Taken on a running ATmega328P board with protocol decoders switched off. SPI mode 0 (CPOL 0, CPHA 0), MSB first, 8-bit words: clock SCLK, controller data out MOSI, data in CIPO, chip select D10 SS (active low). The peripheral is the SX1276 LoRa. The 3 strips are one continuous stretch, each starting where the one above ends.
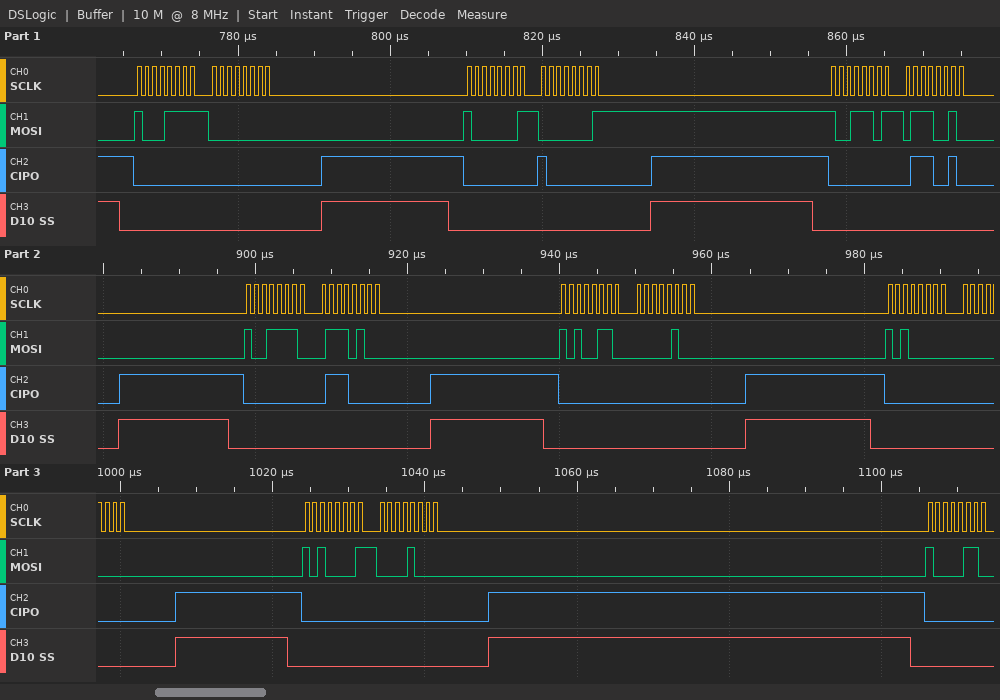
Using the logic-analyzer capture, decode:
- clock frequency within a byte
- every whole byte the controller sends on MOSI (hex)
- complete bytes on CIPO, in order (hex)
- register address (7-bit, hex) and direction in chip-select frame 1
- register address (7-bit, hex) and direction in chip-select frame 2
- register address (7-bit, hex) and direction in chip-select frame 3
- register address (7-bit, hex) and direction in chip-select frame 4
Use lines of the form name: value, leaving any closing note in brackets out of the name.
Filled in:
clock frequency within a byte: 1 MHz
every whole byte the controller sends on MOSI: 8F 00 81 01 9D 72 9E 74 A6 04 A0 00 A1 08 86
complete bytes on CIPO, in order: 00 00 00 80 00 72 00 70 00 00 00 00 00 00 00
register address (7-bit, hex) and direction in chip-select frame 1: 0x0F write
register address (7-bit, hex) and direction in chip-select frame 2: 0x01 write
register address (7-bit, hex) and direction in chip-select frame 3: 0x1D write
register address (7-bit, hex) and direction in chip-select frame 4: 0x1E write
